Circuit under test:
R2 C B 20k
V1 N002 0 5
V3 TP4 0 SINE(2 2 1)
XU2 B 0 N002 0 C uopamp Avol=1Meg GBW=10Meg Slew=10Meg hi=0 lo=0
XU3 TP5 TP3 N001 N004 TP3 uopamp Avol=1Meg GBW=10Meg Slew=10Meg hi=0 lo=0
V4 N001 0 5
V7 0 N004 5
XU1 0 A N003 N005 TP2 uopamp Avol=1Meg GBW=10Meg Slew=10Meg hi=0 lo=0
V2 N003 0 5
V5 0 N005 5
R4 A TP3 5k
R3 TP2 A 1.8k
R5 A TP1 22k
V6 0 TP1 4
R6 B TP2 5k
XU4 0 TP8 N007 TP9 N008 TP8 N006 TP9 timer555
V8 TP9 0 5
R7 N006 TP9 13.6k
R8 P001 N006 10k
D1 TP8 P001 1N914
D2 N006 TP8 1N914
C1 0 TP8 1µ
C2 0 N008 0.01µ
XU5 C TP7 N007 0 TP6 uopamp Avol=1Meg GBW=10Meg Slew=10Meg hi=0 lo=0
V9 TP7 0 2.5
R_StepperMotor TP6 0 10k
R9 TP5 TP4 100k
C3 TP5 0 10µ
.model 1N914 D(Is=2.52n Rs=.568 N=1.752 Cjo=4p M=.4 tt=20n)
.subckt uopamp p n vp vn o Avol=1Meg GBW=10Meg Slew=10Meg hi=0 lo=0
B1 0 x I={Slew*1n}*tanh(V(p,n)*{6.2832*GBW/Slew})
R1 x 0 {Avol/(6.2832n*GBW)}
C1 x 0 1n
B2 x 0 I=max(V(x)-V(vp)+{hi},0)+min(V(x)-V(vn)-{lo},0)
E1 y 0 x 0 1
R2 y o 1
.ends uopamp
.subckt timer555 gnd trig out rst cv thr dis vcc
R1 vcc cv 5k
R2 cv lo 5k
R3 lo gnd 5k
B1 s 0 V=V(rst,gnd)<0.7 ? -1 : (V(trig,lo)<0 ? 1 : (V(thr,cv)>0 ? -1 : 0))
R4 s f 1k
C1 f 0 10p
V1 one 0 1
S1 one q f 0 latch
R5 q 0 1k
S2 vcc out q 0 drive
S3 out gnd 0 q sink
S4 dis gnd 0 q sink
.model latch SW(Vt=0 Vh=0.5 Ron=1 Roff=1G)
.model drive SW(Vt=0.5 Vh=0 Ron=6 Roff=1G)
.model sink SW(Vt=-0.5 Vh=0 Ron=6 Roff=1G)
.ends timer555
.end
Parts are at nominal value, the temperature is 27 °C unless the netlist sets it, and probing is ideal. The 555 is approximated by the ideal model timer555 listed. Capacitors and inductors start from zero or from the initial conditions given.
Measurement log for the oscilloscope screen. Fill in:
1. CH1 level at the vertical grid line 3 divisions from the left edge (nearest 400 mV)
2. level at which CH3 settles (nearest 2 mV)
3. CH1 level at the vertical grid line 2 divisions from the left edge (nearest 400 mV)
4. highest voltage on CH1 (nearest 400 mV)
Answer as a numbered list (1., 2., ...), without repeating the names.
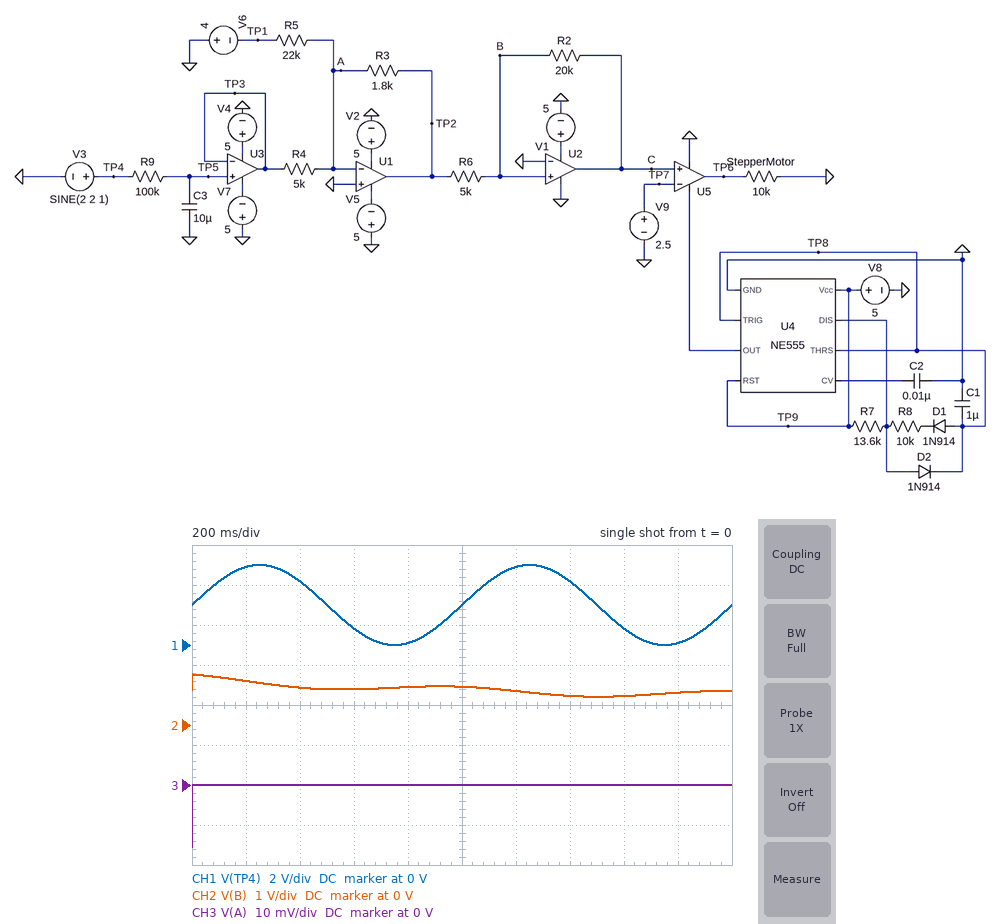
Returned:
1. 800 mV
2. 0 V
3. 3.2 V
4. 4.0 V
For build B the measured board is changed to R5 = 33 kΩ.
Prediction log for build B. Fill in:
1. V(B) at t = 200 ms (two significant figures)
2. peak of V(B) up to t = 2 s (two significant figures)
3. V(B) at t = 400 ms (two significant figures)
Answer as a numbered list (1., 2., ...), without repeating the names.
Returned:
1. 1.0 V
2. 1.2 V
3. 850 mV
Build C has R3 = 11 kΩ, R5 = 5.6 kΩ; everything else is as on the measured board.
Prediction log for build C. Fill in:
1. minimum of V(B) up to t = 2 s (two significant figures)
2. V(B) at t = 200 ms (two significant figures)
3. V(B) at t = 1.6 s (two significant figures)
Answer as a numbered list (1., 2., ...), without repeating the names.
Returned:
1. 3.9 V
2. 5.0 V
3. 4.0 V
